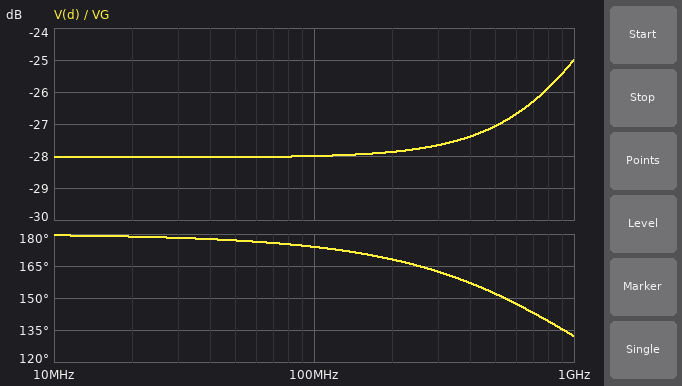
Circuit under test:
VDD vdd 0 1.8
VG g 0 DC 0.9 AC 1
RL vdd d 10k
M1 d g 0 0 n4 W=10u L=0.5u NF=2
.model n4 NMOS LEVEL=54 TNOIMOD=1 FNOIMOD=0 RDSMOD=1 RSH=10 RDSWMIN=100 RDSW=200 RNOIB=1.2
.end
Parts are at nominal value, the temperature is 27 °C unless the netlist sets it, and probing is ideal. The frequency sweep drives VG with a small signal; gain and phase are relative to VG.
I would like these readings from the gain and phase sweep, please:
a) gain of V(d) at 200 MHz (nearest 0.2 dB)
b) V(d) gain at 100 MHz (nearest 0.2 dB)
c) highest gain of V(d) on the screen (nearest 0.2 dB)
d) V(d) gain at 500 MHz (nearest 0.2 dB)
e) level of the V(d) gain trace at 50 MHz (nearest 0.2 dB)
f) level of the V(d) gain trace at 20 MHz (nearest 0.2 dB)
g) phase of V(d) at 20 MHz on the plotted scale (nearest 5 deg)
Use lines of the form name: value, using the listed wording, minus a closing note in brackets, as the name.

gain of V(d) at 200 MHz: -27.8 dB
V(d) gain at 100 MHz: -28.0 dB
highest gain of V(d) on the screen: -25.0 dB
V(d) gain at 500 MHz: -27.0 dB
level of the V(d) gain trace at 50 MHz: -28.0 dB
level of the V(d) gain trace at 20 MHz: -28.0 dB
phase of V(d) at 20 MHz on the plotted scale: 180 deg
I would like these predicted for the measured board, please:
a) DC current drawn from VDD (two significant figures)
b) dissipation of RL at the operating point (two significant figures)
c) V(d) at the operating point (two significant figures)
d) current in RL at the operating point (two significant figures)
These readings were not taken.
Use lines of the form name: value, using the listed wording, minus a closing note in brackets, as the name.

DC current drawn from VDD: 180 µA
dissipation of RL at the operating point: 310 µW
V(d) at the operating point: 30 mV
current in RL at the operating point: 180 µA
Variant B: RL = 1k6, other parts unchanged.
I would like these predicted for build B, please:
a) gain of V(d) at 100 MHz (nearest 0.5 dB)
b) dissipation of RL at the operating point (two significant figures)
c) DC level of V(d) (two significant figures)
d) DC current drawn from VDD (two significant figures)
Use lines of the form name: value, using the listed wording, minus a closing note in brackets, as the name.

gain of V(d) at 100 MHz: -8.0 dB
dissipation of RL at the operating point: 1.6 mW
DC level of V(d): 210 mV
DC current drawn from VDD: 990 µA
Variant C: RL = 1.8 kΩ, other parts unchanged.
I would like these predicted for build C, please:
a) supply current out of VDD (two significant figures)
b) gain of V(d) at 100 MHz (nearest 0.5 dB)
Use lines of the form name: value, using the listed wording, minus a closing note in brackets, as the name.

supply current out of VDD: 900 µA
gain of V(d) at 100 MHz: -9.5 dB
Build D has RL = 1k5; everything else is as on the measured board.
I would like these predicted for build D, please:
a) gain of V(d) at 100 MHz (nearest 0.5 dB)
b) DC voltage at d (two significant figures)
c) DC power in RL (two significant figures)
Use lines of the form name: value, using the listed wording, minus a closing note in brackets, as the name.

gain of V(d) at 100 MHz: -7.0 dB
DC voltage at d: 230 mV
DC power in RL: 1.6 mW
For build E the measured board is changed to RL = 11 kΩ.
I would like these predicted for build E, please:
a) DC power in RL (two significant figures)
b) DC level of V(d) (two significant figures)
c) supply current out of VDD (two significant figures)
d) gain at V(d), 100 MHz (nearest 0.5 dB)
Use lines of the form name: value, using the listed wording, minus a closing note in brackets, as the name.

DC power in RL: 290 µW
DC level of V(d): 27 mV
supply current out of VDD: 160 µA
gain at V(d), 100 MHz: -29.0 dB
